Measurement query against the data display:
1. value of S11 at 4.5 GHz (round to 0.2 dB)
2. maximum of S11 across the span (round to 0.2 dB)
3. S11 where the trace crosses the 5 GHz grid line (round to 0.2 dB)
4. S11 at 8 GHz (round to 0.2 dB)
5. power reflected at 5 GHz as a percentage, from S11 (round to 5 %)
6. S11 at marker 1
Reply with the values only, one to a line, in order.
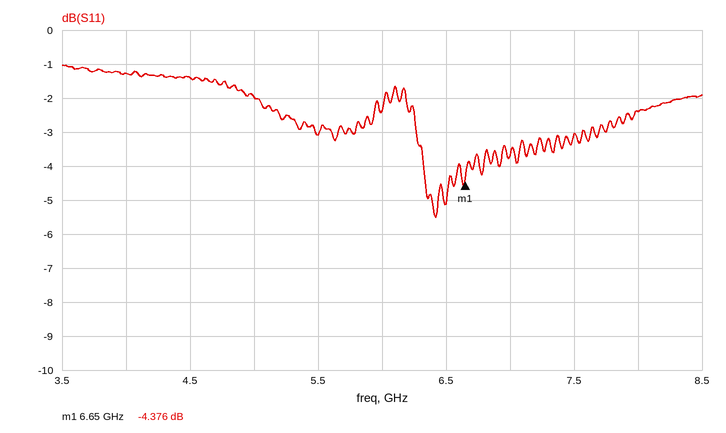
-1.4 dB
-1.0 dB
-2.0 dB
-2.4 dB
65 %
-4.376 dB
